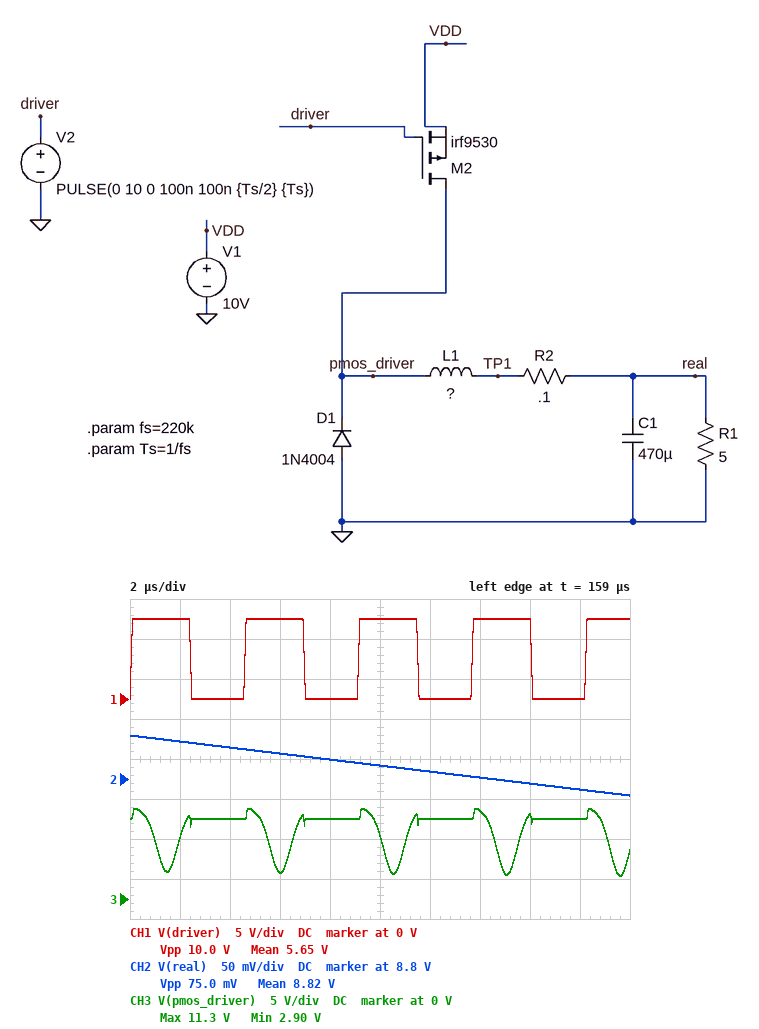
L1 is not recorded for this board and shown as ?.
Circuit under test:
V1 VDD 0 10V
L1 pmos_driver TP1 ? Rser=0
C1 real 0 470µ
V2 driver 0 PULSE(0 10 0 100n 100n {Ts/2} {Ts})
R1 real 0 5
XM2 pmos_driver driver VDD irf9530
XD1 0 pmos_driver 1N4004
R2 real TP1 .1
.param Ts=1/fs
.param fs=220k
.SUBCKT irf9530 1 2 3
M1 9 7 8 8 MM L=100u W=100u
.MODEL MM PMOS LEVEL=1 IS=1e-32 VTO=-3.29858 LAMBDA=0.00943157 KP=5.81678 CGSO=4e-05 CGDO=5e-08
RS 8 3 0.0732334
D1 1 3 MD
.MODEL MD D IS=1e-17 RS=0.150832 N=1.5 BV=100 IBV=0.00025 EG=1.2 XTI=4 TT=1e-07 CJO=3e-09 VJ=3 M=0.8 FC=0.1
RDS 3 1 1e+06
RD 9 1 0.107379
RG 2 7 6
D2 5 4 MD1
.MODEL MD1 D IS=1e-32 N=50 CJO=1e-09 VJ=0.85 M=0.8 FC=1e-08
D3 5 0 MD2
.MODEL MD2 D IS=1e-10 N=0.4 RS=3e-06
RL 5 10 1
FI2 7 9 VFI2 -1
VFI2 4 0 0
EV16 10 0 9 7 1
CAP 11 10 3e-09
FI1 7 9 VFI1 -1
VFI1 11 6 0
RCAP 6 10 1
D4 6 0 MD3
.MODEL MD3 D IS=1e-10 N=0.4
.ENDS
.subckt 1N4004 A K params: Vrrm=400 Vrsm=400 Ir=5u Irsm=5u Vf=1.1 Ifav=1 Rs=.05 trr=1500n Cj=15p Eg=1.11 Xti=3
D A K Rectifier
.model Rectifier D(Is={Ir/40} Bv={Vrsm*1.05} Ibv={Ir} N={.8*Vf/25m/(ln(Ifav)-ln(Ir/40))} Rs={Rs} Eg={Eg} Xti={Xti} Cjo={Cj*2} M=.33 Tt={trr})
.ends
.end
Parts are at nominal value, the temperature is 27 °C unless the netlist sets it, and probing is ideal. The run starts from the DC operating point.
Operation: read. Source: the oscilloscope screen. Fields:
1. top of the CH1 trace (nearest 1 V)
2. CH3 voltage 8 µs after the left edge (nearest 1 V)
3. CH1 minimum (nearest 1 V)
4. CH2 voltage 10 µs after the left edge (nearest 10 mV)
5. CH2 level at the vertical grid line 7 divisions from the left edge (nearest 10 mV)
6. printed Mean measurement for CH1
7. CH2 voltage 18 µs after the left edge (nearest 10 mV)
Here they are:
10 V
10 V
0 V
8.82 V
8.80 V
5.65 V
8.79 V
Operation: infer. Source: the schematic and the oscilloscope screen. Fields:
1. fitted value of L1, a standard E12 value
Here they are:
82 µH
